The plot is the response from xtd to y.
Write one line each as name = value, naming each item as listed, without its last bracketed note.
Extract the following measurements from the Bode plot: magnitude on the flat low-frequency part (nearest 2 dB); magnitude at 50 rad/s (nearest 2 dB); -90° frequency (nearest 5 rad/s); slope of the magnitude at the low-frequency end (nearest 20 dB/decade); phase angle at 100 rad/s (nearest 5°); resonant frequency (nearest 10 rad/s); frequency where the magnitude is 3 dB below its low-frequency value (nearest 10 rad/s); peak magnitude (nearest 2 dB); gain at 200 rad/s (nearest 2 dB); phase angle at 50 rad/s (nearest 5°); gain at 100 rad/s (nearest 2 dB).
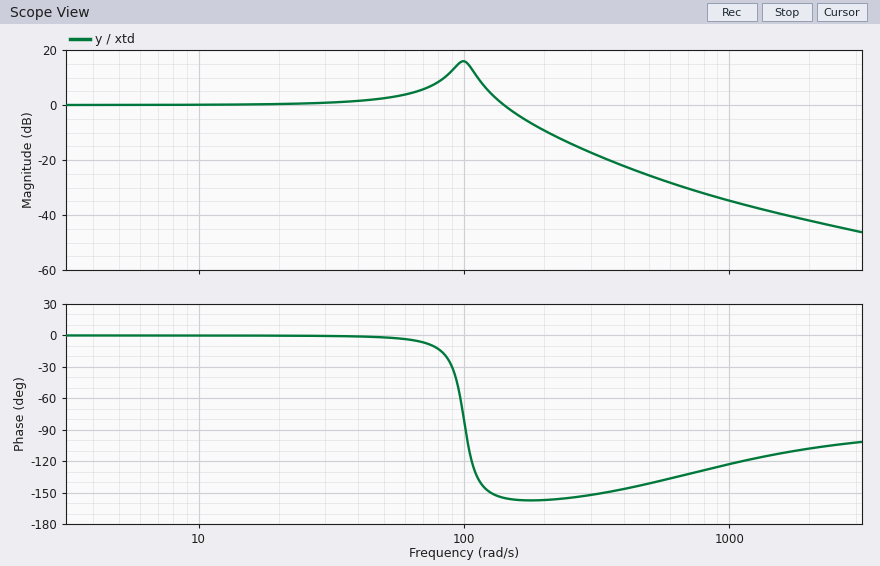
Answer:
magnitude on the flat low-frequency part = 0 dB
magnitude at 50 rad/s = 2 dB
-90° frequency = 100 rad/s
slope of the magnitude at the low-frequency end = 0 dB/decade
phase angle at 100 rad/s = -80°
resonant frequency = 100 rad/s
frequency where the magnitude is 3 dB below its low-frequency value = 160 rad/s
peak magnitude = 16 dB
gain at 200 rad/s = -10 dB
phase angle at 50 rad/s = 0°
gain at 100 rad/s = 16 dB
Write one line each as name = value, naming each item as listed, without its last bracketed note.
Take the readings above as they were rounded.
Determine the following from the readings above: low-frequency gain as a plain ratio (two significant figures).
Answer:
low-frequency gain as a plain ratio = 1.0
